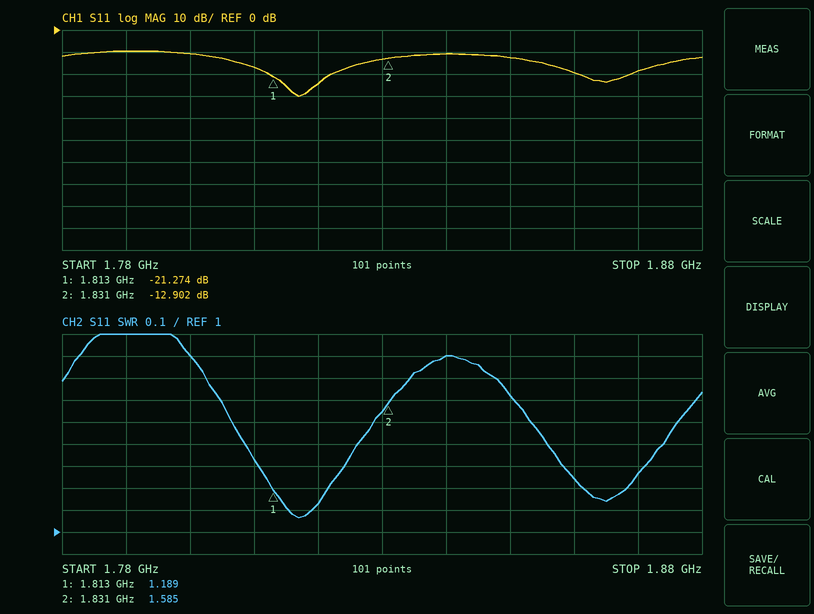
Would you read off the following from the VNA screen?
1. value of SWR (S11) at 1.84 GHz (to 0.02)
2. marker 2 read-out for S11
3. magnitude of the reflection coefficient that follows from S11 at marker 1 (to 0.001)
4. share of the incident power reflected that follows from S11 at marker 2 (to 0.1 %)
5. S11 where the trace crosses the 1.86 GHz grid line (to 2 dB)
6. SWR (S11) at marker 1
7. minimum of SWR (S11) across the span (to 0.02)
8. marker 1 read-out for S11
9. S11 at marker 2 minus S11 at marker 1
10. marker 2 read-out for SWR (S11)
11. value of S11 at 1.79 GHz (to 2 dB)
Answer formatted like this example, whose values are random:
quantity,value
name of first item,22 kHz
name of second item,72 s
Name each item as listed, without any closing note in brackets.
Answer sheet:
quantity,value
value of SWR (S11) at 1.84 GHz,1.80
marker 2 read-out for S11,-12.902 dB
magnitude of the reflection coefficient that follows from S11 at marker 1,0.086
share of the incident power reflected that follows from S11 at marker 2,5.1 %
S11 where the trace crosses the 1.86 GHz grid line,-20 dB
SWR (S11) at marker 1,1.189
minimum of SWR (S11) across the span,1.06
marker 1 read-out for S11,-21.274 dB
S11 at marker 2 minus S11 at marker 1,8.372 dB
marker 2 read-out for SWR,1.585
value of S11 at 1.79 GHz,-10 dB
